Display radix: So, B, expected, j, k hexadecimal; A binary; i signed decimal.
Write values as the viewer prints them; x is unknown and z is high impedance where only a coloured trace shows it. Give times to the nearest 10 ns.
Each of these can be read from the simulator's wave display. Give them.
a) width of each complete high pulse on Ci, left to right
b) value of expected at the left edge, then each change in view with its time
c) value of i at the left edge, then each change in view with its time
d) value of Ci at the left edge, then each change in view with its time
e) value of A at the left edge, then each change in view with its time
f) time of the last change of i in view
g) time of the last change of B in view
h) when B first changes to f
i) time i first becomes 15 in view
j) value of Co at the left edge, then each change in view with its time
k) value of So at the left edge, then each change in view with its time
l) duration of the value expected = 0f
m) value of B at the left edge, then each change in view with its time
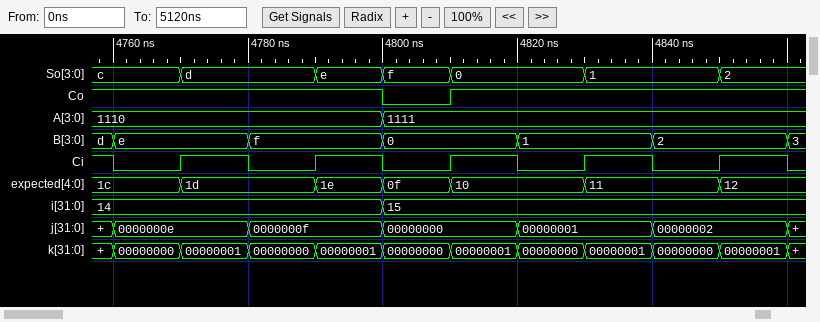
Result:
10 ns, 10 ns, 10 ns, 10 ns, 10 ns
1c, 1d at 4770 ns, 1e at 4790 ns, 0f at 4800 ns, 10 at 4810 ns, 11 at 4830 ns, 12 at 4850 ns
14, 15 at 4800 ns
1, 0 at 4760 ns, 1 at 4770 ns, 0 at 4780 ns, 1 at 4790 ns, 0 at 4800 ns, 1 at 4810 ns, 0 at 4820 ns, 1 at 4830 ns, 0 at 4840 ns, 1 at 4850 ns, 0 at 4860 ns
1110, 1111 at 4800 ns
4800 ns
4860 ns
4780 ns
4800 ns
1, 0 at 4800 ns, 1 at 4810 ns
c, d at 4770 ns, e at 4790 ns, f at 4800 ns, 0 at 4810 ns, 1 at 4830 ns, 2 at 4850 ns
10 ns
d, e at 4760 ns, f at 4780 ns, 0 at 4800 ns, 1 at 4820 ns, 2 at 4840 ns, 3 at 4860 ns
